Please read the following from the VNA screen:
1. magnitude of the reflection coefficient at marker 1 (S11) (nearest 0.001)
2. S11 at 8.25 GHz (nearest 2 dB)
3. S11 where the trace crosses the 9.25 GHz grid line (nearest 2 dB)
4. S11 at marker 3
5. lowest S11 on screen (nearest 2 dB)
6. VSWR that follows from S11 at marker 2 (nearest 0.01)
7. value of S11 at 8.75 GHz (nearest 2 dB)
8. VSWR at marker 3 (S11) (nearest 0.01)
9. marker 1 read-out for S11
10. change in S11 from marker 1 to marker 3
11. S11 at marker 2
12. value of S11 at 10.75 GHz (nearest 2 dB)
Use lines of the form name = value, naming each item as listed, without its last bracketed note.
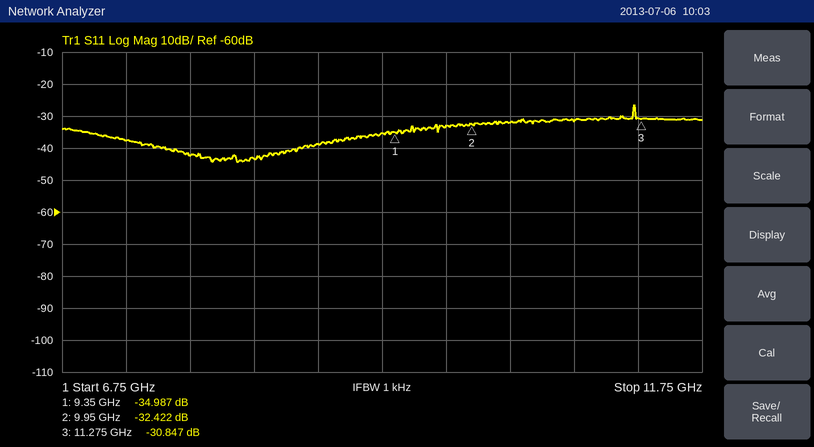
magnitude of the reflection coefficient at marker 1 (S11) = 0.018
S11 at 8.25 GHz = -44 dB
S11 where the trace crosses the 9.25 GHz grid line = -36 dB
S11 at marker 3 = -30.847 dB
lowest S11 on screen = -44 dB
VSWR that follows from S11 at marker 2 = 1.05
value of S11 at 8.75 GHz = -38 dB
VSWR at marker 3 (S11) = 1.06
marker 1 read-out for S11 = -34.987 dB
change in S11 from marker 1 to marker 3 = 4.140 dB
S11 at marker 2 = -32.422 dB
value of S11 at 10.75 GHz = -32 dB
